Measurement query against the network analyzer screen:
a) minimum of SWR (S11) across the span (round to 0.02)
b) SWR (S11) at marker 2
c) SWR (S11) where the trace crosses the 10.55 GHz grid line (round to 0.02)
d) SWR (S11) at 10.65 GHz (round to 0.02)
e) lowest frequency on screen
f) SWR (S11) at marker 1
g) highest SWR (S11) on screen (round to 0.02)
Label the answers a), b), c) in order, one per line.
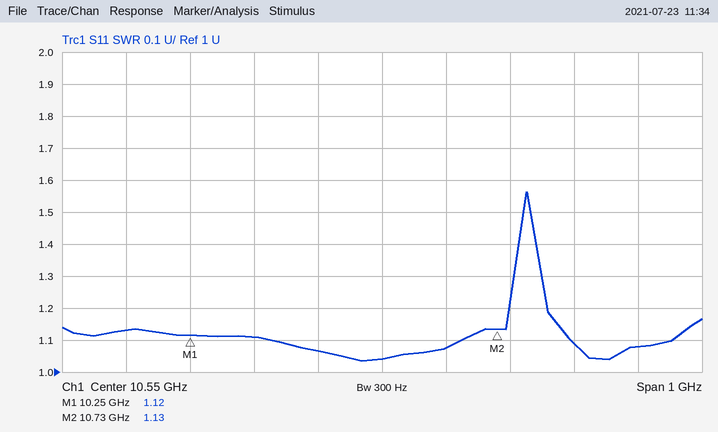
a) 1.04
b) 1.13
c) 1.04
d) 1.08
e) 10.05 GHz
f) 1.12
g) 1.56
